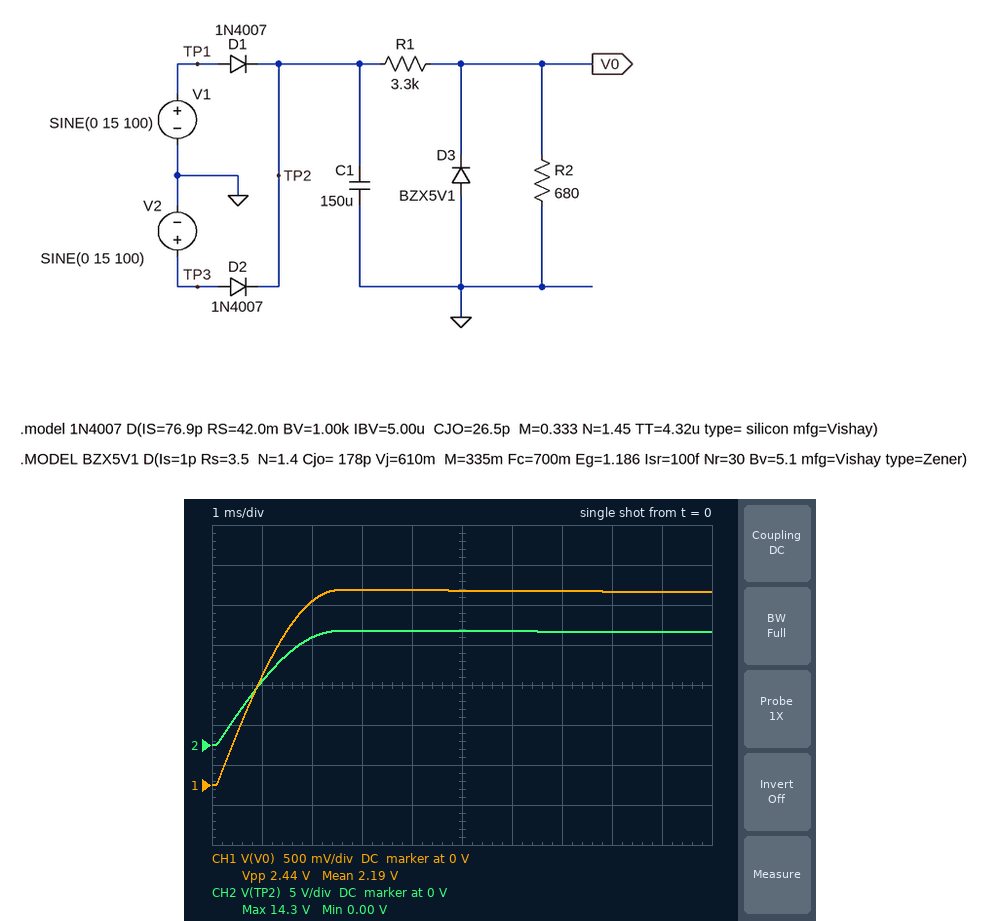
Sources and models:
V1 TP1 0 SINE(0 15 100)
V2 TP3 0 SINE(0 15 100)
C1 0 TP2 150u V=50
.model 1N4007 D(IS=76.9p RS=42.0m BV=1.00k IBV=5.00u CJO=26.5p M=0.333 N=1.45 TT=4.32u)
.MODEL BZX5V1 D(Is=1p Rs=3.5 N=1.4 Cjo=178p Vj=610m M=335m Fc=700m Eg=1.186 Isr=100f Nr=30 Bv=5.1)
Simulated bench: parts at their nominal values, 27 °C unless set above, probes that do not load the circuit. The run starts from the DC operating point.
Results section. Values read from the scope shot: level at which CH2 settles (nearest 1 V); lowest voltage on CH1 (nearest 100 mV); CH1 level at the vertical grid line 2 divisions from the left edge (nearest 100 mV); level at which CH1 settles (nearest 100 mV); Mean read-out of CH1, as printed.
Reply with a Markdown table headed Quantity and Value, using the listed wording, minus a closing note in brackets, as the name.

| Quantity | Value |
|---|---|
| level at which CH2 settles | 14 V |
| lowest voltage on CH1 | 0 V |
| CH1 level at the vertical grid line 2 divisions from the left edge | 2.3 V |
| level at which CH1 settles | 2.4 V |
| Mean read-out of CH1, as printed | 2.19 V |
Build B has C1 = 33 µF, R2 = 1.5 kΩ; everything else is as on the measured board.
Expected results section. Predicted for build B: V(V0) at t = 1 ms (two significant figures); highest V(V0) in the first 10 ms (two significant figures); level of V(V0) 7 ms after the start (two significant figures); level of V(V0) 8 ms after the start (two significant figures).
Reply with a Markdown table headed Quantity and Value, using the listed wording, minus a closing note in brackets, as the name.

| Quantity | Value |
|---|---|
| V(V0) at t = 1 ms | 2.5 V |
| highest V(V0) in the first 10 ms | 4.5 V |
| level of V(V0) 7 ms after the start | 4.4 V |
| level of V(V0) 8 ms after the start | 4.3 V |
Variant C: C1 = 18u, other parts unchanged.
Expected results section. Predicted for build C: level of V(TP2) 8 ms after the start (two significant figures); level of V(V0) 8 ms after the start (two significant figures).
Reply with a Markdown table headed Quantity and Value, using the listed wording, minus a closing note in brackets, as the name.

| Quantity | Value |
|---|---|
| level of V(TP2) 8 ms after the start | 13 V |
| level of V(V0) 8 ms after the start | 2.3 V |
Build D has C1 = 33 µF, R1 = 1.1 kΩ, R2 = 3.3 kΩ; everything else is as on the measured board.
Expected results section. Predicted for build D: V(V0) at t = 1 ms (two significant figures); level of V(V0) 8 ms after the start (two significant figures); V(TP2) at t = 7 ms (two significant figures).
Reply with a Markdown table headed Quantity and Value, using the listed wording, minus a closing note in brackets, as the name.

| Quantity | Value |
|---|---|
| V(V0) at t = 1 ms | 5.1 V |
| level of V(V0) 8 ms after the start | 5.2 V |
| V(TP2) at t = 7 ms | 13 V |
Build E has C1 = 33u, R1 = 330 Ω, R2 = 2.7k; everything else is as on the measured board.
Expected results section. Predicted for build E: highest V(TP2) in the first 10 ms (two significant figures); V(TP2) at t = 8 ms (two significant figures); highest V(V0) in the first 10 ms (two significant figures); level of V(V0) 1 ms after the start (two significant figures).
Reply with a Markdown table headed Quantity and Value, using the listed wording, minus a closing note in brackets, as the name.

| Quantity | Value |
|---|---|
| highest V(TP2) in the first 10 ms | 14 V |
| V(TP2) at t = 8 ms | 11 V |
| highest V(V0) in the first 10 ms | 5.3 V |
| level of V(V0) 1 ms after the start | 5.2 V |
